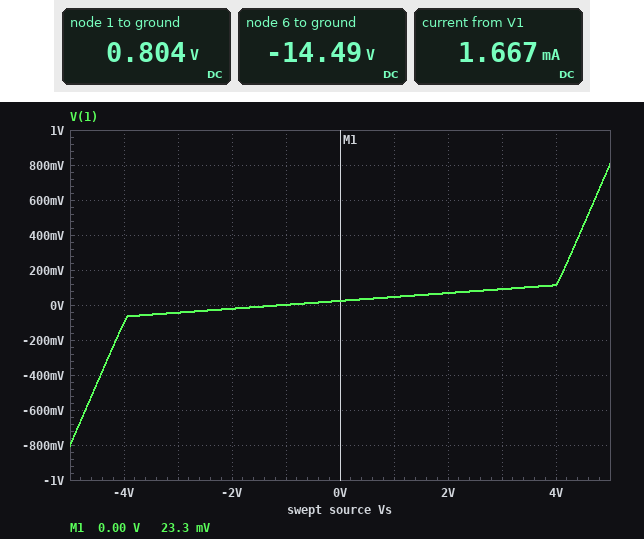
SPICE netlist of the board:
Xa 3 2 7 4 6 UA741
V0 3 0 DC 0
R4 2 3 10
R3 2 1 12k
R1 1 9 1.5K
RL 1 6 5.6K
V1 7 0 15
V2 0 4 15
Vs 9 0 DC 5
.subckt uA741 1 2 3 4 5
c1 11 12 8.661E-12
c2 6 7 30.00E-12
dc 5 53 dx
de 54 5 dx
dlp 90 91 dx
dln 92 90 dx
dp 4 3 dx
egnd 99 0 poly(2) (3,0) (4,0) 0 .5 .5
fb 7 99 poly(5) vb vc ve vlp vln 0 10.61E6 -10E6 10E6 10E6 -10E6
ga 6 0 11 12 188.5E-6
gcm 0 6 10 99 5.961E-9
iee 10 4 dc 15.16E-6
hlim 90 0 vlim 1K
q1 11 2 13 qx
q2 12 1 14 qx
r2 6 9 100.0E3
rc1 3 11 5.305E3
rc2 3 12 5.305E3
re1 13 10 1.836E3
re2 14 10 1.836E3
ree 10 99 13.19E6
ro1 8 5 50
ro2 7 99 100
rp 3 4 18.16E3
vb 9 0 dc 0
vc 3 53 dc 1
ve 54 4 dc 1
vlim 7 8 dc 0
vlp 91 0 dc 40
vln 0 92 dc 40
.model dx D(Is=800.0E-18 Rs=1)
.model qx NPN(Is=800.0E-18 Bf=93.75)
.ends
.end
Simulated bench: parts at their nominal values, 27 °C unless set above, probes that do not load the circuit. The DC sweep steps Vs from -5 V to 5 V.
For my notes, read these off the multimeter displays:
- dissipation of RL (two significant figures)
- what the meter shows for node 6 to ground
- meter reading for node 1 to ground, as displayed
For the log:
42 mW
-14.49 V
0.804 V
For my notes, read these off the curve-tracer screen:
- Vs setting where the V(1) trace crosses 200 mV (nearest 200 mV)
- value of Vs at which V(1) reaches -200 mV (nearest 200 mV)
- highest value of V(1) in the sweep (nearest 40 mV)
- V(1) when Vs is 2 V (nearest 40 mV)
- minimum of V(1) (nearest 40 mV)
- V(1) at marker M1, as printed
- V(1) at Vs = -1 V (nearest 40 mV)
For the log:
4.2 V
-4.2 V
800 mV
80 mV
-800 mV
23.3 mV
0 V
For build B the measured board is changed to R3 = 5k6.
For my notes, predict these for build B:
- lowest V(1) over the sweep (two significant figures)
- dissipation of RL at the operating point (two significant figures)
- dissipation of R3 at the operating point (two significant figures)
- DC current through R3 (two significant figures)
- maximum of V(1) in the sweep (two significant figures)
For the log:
-730 mV
41 mW
94 µW
130 µA
730 mV
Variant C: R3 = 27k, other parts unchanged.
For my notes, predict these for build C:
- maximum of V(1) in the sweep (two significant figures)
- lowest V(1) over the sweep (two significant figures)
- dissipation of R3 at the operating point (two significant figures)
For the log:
850 mV
-850 mV
27 µW
